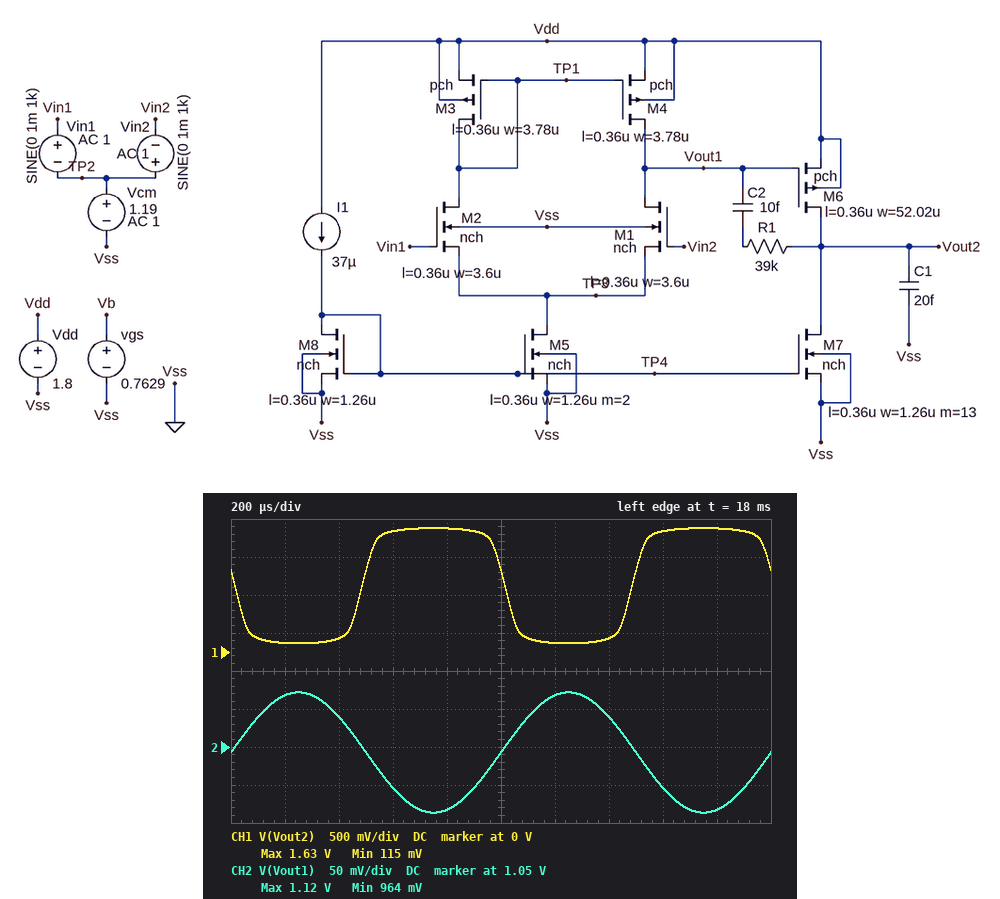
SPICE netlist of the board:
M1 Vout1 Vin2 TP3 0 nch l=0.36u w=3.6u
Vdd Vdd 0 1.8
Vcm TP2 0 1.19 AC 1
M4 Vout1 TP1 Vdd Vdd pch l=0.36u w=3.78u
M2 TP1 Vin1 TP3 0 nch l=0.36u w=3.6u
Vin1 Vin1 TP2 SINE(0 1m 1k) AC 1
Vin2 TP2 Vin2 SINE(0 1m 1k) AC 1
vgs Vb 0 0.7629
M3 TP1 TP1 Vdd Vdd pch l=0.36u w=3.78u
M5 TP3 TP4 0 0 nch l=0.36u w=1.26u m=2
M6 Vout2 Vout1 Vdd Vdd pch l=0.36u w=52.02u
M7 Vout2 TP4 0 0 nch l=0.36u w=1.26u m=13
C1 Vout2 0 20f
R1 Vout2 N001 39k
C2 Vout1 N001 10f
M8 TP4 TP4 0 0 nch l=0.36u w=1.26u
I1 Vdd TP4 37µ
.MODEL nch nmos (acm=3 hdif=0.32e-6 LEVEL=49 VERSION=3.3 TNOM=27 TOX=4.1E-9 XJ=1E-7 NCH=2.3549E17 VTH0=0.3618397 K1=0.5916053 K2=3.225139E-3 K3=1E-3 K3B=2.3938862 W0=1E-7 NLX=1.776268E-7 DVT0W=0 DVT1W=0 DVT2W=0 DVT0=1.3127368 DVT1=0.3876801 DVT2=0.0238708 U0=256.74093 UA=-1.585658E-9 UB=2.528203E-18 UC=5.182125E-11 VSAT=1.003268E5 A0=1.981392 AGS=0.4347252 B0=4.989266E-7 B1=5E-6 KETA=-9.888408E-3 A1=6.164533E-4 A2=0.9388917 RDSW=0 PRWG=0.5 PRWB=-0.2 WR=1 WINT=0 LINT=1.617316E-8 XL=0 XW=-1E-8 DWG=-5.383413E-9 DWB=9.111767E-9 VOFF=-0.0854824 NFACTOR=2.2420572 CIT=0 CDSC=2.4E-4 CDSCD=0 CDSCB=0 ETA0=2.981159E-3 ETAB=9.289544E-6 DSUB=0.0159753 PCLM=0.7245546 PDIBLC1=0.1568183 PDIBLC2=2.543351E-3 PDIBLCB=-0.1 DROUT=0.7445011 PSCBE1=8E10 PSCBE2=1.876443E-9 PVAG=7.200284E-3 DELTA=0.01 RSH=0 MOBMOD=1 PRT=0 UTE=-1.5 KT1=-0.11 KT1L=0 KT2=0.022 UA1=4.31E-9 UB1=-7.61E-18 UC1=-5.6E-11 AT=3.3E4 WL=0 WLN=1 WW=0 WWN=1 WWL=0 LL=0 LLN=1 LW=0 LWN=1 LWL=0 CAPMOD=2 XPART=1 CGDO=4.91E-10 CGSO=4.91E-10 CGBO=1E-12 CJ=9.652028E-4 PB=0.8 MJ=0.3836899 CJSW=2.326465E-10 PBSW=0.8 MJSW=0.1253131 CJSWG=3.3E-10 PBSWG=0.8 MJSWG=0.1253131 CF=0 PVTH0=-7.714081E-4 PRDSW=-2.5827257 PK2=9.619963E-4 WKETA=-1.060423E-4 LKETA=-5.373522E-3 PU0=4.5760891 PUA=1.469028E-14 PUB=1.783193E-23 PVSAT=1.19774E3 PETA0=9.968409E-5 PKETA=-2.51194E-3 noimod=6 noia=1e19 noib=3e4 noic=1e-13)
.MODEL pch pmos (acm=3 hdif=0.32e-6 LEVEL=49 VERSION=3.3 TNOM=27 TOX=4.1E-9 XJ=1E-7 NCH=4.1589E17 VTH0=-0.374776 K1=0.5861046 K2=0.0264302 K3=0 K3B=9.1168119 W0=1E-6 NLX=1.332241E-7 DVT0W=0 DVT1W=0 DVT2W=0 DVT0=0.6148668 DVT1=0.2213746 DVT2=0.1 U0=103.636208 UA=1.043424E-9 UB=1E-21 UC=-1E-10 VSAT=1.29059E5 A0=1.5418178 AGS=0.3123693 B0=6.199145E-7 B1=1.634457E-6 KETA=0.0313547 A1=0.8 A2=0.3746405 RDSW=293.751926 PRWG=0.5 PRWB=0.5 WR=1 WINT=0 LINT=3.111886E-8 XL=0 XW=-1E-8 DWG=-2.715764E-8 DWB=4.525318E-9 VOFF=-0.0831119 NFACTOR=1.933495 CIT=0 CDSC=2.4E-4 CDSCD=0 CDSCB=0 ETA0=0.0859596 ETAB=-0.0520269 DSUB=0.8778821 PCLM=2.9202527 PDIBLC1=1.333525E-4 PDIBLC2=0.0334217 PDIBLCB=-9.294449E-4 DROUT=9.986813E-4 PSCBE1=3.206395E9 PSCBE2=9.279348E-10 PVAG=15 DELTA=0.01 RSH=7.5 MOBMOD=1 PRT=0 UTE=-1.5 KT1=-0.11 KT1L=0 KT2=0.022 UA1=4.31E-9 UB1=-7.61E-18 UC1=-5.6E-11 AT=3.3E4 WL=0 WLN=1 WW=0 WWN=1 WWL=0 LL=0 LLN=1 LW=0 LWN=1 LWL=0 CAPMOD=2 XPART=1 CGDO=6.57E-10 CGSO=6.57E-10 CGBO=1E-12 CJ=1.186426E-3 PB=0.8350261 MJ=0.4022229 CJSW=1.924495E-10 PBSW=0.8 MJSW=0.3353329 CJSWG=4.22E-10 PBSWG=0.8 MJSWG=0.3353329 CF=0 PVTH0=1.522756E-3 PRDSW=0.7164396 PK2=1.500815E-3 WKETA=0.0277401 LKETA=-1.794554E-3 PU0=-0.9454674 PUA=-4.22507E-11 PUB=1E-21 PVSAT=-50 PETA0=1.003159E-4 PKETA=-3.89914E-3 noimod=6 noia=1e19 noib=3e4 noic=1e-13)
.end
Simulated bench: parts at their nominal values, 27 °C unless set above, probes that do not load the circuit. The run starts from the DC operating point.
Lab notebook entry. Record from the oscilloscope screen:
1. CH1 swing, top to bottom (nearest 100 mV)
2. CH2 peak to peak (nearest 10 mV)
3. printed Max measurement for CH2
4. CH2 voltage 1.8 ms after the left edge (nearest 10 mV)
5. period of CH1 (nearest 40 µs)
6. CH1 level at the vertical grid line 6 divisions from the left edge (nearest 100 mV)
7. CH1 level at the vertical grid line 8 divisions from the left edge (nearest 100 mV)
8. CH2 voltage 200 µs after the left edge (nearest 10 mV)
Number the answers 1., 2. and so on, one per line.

1. 1.5 V
2. 160 mV
3. 1.12 V
4. 970 mV
5. 1.00 ms
6. 100 mV
7. 1.6 V
8. 1.12 V
